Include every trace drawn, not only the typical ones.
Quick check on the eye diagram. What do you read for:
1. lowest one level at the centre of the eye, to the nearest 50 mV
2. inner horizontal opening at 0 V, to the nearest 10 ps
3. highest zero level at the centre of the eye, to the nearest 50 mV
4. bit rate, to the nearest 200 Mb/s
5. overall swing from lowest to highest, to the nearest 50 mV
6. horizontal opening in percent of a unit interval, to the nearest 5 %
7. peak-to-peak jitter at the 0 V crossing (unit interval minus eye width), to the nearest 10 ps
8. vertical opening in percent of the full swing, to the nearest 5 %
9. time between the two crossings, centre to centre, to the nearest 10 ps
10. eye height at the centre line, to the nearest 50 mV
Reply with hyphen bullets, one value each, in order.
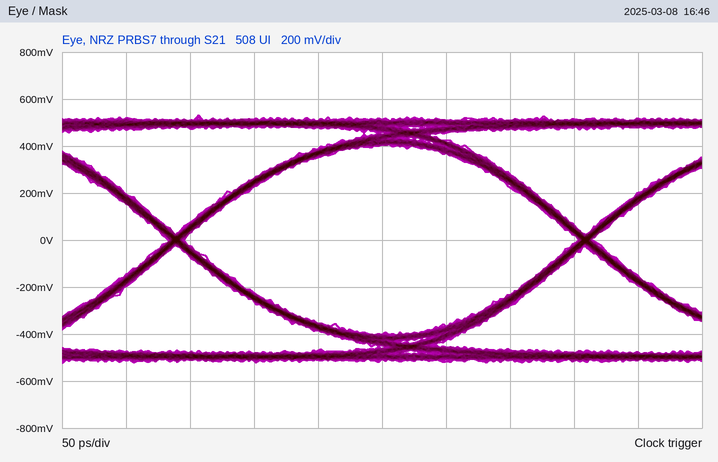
- 400 mV
- 310 ps
- -400 mV
- 3.2 Gb/s
- 1.05 V
- 95 %
- 10 ps
- 75 %
- 320 ps
- 800 mV
